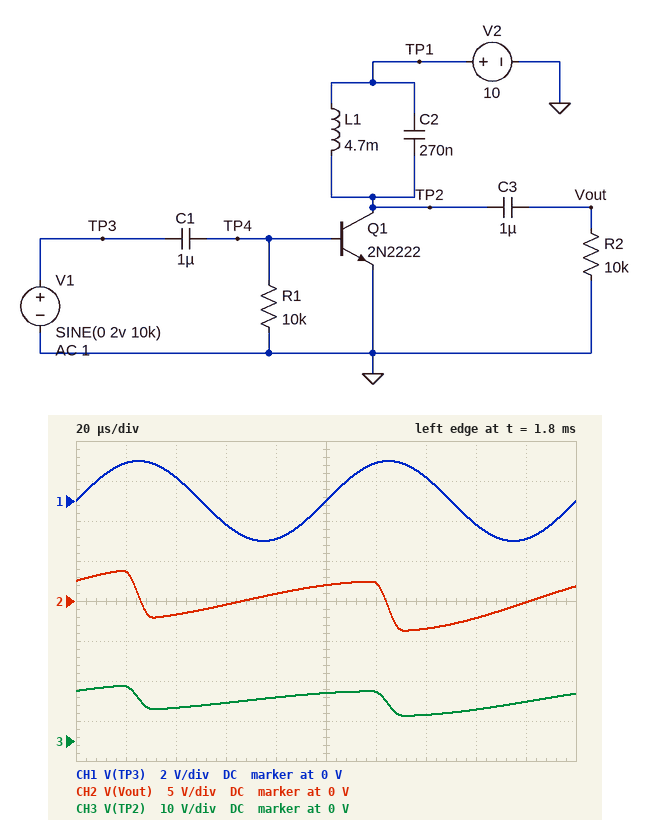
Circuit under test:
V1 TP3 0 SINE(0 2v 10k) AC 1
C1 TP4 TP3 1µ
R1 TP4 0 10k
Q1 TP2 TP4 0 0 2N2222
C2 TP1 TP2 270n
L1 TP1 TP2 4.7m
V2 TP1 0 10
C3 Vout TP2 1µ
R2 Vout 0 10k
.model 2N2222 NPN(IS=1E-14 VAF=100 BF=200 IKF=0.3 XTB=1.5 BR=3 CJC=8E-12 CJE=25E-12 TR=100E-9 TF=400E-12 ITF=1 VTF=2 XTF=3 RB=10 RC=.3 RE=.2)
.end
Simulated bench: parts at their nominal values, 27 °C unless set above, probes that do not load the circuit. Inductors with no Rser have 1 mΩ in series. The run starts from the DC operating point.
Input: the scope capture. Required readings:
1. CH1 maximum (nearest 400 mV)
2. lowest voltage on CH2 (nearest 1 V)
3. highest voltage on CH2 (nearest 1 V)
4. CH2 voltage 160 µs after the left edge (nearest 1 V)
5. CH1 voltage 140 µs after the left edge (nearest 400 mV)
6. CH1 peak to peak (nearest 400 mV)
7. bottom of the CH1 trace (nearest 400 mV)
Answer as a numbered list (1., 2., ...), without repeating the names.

1. 2.0 V
2. -4 V
3. 4 V
4. -2 V
5. 1.2 V
6. 4.0 V
7. -2.0 V
